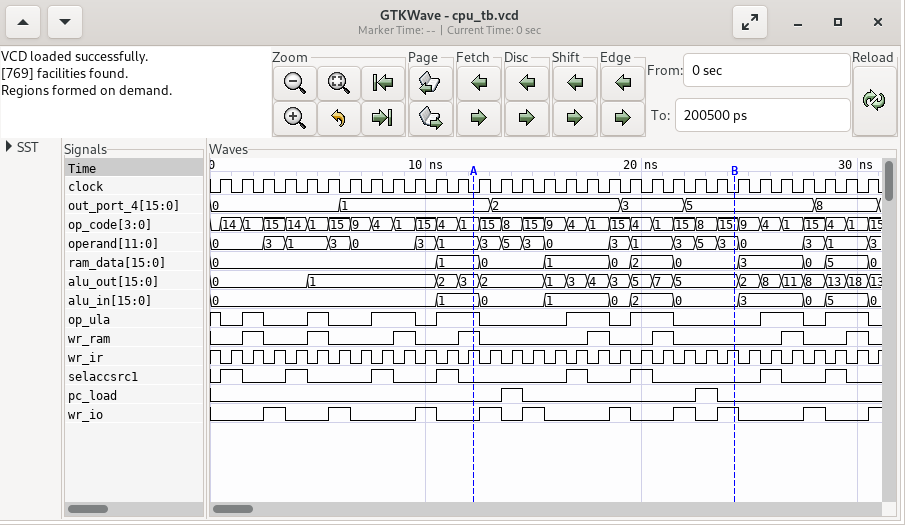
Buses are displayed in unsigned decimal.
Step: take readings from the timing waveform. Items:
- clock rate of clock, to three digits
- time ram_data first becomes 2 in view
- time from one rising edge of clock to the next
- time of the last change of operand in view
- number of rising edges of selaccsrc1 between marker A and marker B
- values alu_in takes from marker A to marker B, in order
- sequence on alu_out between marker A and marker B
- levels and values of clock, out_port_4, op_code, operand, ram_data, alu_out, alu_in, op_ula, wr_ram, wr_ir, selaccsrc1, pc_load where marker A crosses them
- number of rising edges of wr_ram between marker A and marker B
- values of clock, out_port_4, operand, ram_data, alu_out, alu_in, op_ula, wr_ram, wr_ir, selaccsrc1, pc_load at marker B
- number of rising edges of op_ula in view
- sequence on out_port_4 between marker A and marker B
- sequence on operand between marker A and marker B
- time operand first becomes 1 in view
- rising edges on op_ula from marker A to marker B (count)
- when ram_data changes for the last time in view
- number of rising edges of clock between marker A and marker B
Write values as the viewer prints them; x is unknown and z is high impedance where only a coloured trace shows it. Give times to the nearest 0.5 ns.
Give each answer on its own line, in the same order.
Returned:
1.00 GHz
19.5 ns
1 ns
30.5 ns
2
1, 0, 1, 0, 2, 0
3, 2, 1, 3, 4, 3, 5, 7, 5
clock=0, out_port_4=1, op_code=1, operand=1, ram_data=1, alu_out=3, alu_in=1, op_ula=1, wr_ram=1, wr_ir=1, selaccsrc1=0, pc_load=0
2
clock=0, out_port_4=5, operand=3, ram_data=0, alu_out=5, alu_in=0, op_ula=0, wr_ram=0, wr_ir=1, selaccsrc1=0, pc_load=0
8
1, 2, 3, 5
1, 3, 5, 3, 0, 3, 1, 3, 5, 3
3.5 ns
2
30.5 ns
12
